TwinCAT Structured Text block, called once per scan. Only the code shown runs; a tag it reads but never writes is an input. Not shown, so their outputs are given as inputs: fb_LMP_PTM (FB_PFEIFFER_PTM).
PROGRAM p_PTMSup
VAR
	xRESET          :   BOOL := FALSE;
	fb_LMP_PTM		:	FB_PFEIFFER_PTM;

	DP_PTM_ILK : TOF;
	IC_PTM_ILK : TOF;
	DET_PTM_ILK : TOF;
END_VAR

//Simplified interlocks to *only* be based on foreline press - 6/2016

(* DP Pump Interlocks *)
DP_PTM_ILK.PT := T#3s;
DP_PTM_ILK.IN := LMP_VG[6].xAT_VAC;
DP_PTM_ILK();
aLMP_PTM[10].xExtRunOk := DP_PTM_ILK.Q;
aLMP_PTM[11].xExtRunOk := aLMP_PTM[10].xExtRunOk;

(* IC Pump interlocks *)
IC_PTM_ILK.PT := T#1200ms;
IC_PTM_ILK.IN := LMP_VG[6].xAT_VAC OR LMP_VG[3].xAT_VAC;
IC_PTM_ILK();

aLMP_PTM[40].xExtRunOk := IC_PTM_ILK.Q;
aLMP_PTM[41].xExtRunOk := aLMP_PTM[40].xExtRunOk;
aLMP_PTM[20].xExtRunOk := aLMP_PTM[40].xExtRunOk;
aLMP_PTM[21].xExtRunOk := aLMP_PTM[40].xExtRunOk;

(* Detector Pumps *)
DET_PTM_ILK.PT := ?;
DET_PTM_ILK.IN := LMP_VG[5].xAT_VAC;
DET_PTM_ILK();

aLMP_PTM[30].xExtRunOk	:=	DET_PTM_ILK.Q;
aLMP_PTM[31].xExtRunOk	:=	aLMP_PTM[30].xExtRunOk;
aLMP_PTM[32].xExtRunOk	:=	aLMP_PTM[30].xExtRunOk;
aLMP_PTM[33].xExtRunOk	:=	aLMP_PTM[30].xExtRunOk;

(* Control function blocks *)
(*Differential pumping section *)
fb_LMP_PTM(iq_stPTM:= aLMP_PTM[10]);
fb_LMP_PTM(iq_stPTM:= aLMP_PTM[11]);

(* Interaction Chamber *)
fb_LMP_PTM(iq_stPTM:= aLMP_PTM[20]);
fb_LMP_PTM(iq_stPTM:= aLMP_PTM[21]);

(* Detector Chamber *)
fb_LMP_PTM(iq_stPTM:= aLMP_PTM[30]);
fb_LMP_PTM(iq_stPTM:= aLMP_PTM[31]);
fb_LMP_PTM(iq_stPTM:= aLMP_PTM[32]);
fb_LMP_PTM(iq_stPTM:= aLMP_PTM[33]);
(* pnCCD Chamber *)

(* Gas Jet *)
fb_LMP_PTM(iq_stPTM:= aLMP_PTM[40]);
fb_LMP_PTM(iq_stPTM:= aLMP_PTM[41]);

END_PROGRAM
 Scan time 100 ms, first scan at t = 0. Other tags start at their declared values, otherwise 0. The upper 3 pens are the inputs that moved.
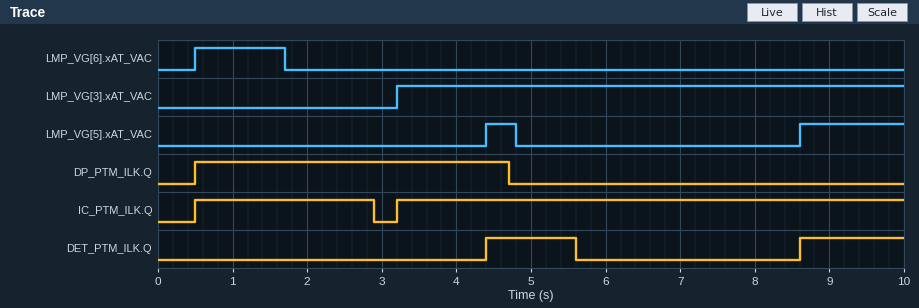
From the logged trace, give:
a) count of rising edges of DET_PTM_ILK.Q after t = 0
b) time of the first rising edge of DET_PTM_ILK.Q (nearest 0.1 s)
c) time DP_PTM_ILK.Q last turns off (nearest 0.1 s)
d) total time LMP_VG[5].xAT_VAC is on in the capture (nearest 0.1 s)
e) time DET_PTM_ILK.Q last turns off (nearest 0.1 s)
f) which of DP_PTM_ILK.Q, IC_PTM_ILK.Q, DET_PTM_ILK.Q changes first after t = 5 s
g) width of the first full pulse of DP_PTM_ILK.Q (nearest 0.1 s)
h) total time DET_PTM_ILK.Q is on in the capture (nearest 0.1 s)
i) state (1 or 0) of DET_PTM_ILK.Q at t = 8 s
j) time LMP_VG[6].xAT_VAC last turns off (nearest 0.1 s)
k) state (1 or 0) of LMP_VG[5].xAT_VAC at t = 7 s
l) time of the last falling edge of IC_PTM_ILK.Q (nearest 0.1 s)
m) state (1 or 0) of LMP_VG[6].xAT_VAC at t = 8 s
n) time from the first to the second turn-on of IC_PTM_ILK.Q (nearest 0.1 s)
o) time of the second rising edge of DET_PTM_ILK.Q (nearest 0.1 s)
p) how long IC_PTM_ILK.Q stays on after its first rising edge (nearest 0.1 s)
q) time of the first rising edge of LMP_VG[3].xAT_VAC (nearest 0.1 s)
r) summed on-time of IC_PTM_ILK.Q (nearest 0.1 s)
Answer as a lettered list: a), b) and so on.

a) 2
b) 4.4 s
c) 4.7 s
d) 1.8 s
e) 5.6 s
f) DET_PTM_ILK.Q
g) 4.2 s
h) 2.6 s
i) 0
j) 1.7 s
k) 0
l) 2.9 s
m) 0
n) 2.7 s
o) 8.6 s
p) 2.4 s
q) 3.2 s
r) 9.2 s
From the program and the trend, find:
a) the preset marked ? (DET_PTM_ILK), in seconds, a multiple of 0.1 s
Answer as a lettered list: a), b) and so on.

a) 0.8 s
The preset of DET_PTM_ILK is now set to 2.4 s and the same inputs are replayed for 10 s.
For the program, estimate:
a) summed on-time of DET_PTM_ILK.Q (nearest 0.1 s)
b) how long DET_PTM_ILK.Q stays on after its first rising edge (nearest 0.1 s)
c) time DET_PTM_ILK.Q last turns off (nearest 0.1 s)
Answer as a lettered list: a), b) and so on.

a) 4.2 s
b) 2.8 s
c) 7.2 s
